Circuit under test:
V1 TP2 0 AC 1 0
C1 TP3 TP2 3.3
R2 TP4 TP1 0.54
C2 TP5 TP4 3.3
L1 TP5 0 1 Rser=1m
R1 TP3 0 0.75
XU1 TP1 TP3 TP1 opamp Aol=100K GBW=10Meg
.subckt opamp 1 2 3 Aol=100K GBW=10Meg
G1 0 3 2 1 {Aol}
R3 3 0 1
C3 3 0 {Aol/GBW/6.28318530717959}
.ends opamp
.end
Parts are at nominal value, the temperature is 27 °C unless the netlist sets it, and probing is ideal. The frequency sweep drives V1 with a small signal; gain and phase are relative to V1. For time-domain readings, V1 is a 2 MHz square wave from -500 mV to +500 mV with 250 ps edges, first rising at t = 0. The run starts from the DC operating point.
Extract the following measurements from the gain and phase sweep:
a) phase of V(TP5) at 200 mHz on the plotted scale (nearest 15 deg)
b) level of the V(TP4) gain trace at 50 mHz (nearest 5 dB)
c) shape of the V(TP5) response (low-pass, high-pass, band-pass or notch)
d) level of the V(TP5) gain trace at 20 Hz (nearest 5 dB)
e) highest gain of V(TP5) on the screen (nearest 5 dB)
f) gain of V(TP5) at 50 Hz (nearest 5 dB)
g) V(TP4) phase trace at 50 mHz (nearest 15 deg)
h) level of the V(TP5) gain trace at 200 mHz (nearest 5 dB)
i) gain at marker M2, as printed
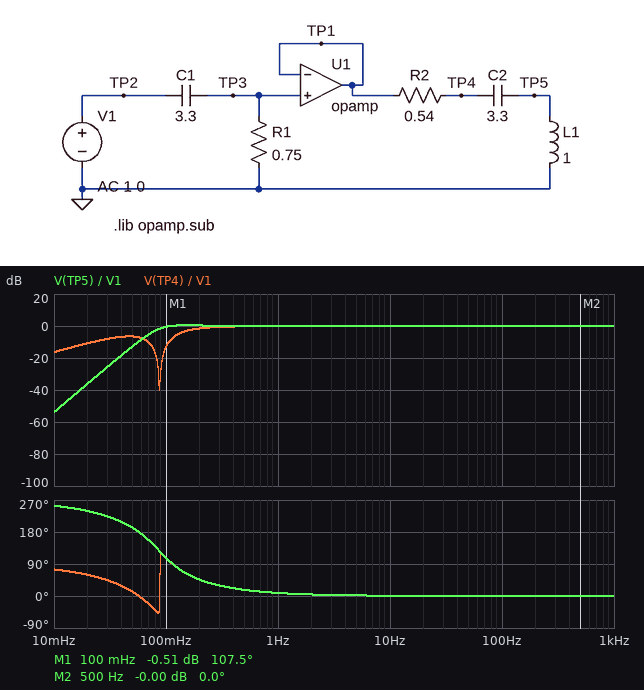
45 deg
-5 dB
high-pass
0 dB
0 dB
0 dB
15 deg
0 dB
-0.00 dB
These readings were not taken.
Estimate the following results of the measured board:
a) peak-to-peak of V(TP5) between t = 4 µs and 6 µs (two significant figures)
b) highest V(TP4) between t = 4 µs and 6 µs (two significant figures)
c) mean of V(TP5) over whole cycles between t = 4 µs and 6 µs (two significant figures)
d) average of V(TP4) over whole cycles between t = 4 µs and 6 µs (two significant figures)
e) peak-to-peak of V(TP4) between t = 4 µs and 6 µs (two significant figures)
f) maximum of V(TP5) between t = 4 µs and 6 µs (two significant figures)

1.0 V
1.0 V
500 mV
500 mV
1.0 V
1.0 V
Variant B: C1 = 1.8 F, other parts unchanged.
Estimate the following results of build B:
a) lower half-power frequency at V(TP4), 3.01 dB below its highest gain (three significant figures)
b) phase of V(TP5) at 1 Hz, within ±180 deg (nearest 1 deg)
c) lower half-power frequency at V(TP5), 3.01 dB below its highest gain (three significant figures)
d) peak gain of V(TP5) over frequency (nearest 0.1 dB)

179 mHz
12 deg
97.7 mHz
0 dB
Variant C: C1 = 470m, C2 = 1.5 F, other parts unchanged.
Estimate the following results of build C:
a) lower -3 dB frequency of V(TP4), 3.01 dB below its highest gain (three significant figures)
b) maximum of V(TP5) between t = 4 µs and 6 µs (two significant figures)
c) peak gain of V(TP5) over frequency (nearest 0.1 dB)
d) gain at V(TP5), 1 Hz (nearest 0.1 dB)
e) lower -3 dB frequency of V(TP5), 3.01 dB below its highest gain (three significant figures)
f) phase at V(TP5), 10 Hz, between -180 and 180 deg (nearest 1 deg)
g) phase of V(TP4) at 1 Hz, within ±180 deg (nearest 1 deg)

470 mHz
1.0 V
0 dB
-0.7 dB
381 mHz
3 deg
29 deg
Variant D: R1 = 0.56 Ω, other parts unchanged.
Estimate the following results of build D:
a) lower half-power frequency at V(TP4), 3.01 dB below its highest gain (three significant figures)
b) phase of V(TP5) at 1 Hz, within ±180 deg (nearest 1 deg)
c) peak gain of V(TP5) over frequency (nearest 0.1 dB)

162 mHz
10 deg
0 dB
